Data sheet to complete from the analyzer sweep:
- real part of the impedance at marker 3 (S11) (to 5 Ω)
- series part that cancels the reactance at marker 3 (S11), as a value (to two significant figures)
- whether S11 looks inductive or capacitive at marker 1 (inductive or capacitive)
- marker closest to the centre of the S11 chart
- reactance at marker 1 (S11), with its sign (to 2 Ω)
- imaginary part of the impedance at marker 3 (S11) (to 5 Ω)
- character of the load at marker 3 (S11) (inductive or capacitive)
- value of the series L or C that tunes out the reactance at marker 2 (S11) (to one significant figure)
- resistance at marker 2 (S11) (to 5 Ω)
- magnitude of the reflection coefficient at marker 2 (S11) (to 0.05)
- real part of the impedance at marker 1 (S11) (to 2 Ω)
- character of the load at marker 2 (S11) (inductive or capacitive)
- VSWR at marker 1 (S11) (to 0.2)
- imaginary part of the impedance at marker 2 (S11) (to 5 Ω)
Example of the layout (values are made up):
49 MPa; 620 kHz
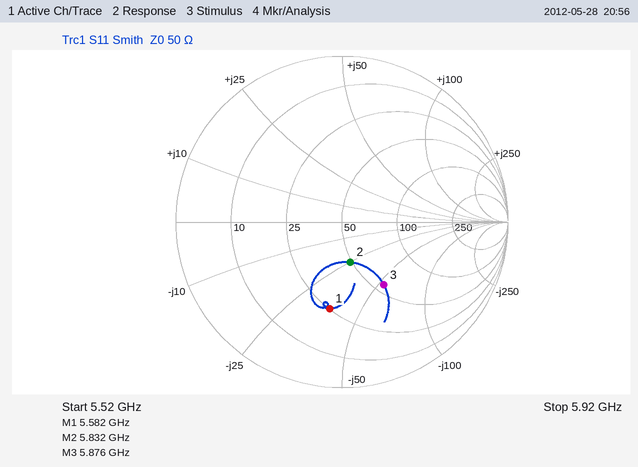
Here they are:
55 Ω; 1.5 nH; capacitive; marker 2; -36 Ω; -55 Ω; capacitive; 700 pH; 50 Ω; 0.25; 26 Ω; capacitive; 3.2; -25 Ω
